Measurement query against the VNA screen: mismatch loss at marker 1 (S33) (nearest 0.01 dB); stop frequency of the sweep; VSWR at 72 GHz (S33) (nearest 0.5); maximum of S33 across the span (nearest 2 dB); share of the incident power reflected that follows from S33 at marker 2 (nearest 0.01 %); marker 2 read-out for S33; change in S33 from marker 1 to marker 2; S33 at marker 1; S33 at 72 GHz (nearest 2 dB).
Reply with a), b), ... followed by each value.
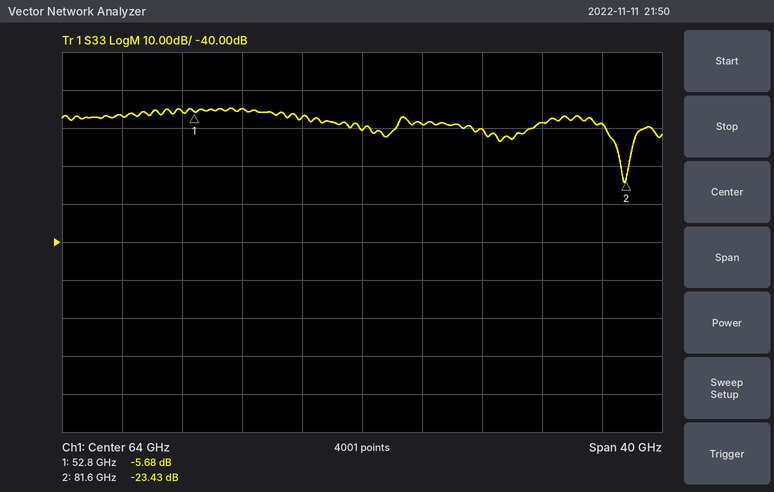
a) 1.37 dB
b) 84 GHz
c) 2.0
d) -4 dB
e) 0.45 %
f) -23.43 dB
g) -17.75 dB
h) -5.68 dB
i) -10 dB
